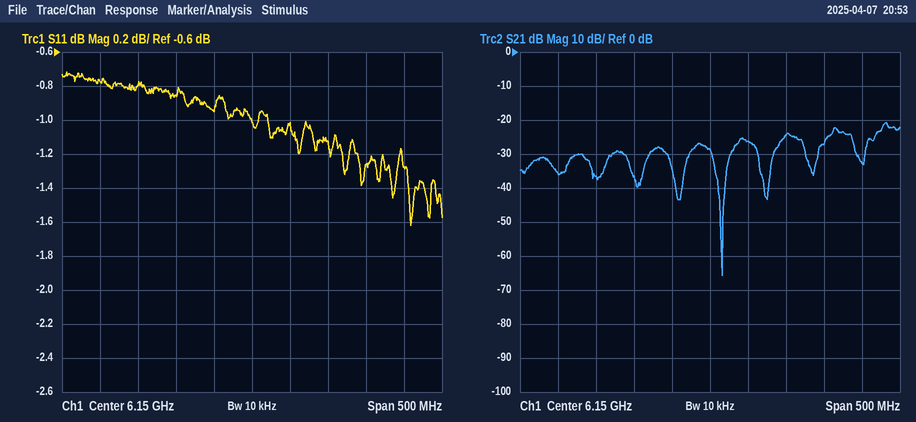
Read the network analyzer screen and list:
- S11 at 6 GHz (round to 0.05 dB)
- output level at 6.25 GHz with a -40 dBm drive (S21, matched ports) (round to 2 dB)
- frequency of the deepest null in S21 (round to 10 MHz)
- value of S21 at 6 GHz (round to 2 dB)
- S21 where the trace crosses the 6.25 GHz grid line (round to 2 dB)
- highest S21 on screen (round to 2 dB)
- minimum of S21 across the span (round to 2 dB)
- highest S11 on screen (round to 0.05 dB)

-0.80 dB
-64 dBm
6.17 GHz
-36 dB
-24 dB
-20 dB
-66 dB
-0.70 dB
